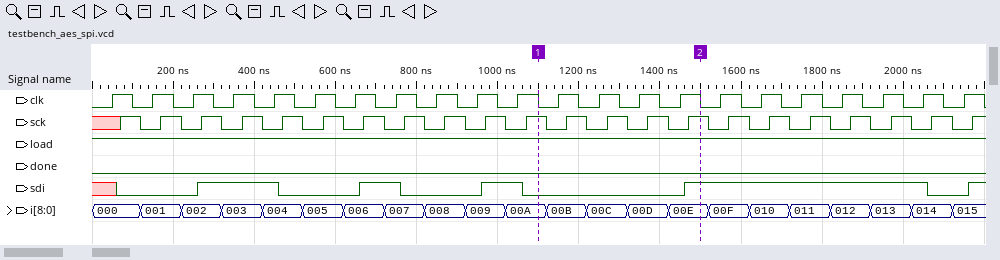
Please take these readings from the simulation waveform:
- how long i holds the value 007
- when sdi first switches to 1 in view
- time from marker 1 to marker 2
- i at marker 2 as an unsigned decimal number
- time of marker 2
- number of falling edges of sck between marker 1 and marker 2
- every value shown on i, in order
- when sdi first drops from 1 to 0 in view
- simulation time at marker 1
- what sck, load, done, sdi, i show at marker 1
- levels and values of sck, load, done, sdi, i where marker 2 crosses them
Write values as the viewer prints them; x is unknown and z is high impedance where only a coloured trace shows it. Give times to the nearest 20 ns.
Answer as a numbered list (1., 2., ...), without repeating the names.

1. 100 ns
2. 260 ns
3. 400 ns
4. 14
5. 1500 ns
6. 4
7. 000, 001, 002, 003, 004, 005, 006, 007, 008, 009, 00A, 00B, 00C, 00D, 00E, 00F, 010, 011, 012, 013, 014, 015
8. 460 ns
9. 1100 ns
10. sck=1, load=1, done=0, sdi=0, i=00A
11. sck=1, load=1, done=0, sdi=1, i=00E
